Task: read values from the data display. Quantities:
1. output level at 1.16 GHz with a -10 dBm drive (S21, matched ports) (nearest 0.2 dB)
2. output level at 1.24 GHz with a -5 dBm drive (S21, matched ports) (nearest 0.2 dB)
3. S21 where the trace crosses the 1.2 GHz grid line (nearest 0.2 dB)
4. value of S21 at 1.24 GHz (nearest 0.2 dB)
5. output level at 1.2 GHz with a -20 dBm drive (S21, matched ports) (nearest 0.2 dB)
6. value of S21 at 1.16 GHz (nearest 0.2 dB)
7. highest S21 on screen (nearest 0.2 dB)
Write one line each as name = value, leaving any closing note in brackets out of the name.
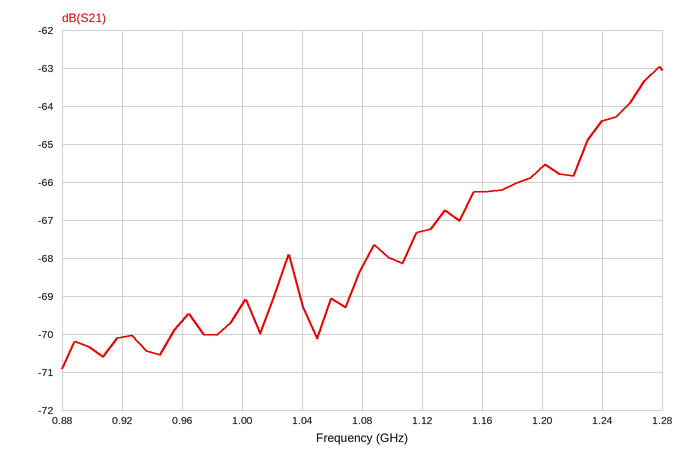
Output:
output level at 1.16 GHz with a -10 dBm drive (S21, matched ports) = -76.2 dBm
output level at 1.24 GHz with a -5 dBm drive (S21, matched ports) = -69.4 dBm
S21 where the trace crosses the 1.2 GHz grid line = -65.6 dB
value of S21 at 1.24 GHz = -64.4 dB
output level at 1.2 GHz with a -20 dBm drive (S21, matched ports) = -85.6 dBm
value of S21 at 1.16 GHz = -66.2 dB
highest S21 on screen = -63.0 dB
